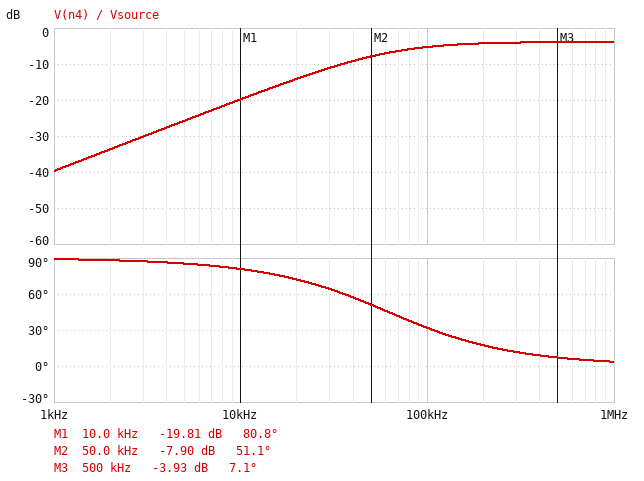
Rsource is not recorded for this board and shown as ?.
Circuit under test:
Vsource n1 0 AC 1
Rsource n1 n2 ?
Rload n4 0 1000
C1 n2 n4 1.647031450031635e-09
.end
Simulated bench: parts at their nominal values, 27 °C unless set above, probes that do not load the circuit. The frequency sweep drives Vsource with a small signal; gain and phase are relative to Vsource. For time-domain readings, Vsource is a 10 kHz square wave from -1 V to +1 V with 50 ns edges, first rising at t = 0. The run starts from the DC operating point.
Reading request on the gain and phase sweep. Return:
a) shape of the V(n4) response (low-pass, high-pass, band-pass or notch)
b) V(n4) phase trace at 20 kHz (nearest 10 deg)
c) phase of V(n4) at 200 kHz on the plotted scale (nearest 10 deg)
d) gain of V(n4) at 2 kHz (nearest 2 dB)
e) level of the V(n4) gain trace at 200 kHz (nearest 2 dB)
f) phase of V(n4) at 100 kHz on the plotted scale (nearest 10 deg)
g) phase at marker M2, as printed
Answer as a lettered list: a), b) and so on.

a) high-pass
b) 70 deg
c) 20 deg
d) -34 dB
e) -4 dB
f) 30 deg
g) 51.1 deg
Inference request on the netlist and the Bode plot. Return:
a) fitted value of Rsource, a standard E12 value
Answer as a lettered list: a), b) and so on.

a) 560 Ω
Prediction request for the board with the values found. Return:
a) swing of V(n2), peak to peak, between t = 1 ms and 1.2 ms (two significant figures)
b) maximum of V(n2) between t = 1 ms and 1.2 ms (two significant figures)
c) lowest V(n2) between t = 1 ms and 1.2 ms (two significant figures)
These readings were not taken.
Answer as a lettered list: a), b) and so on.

a) 2.0 V
b) 1.0 V
c) -1.0 V
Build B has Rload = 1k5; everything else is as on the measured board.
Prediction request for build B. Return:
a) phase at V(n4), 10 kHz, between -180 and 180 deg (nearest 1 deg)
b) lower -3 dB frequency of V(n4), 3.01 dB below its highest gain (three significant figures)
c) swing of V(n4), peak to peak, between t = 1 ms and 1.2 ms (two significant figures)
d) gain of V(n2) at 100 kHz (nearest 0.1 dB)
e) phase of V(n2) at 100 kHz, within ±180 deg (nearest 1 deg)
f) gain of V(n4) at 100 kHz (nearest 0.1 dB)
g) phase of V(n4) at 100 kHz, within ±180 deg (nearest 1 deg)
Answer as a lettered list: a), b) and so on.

a) 78 deg
b) 46.9 kHz
c) 2.9 V
d) -2.1 dB
e) -8 deg
f) -3.6 dB
g) 25 deg
